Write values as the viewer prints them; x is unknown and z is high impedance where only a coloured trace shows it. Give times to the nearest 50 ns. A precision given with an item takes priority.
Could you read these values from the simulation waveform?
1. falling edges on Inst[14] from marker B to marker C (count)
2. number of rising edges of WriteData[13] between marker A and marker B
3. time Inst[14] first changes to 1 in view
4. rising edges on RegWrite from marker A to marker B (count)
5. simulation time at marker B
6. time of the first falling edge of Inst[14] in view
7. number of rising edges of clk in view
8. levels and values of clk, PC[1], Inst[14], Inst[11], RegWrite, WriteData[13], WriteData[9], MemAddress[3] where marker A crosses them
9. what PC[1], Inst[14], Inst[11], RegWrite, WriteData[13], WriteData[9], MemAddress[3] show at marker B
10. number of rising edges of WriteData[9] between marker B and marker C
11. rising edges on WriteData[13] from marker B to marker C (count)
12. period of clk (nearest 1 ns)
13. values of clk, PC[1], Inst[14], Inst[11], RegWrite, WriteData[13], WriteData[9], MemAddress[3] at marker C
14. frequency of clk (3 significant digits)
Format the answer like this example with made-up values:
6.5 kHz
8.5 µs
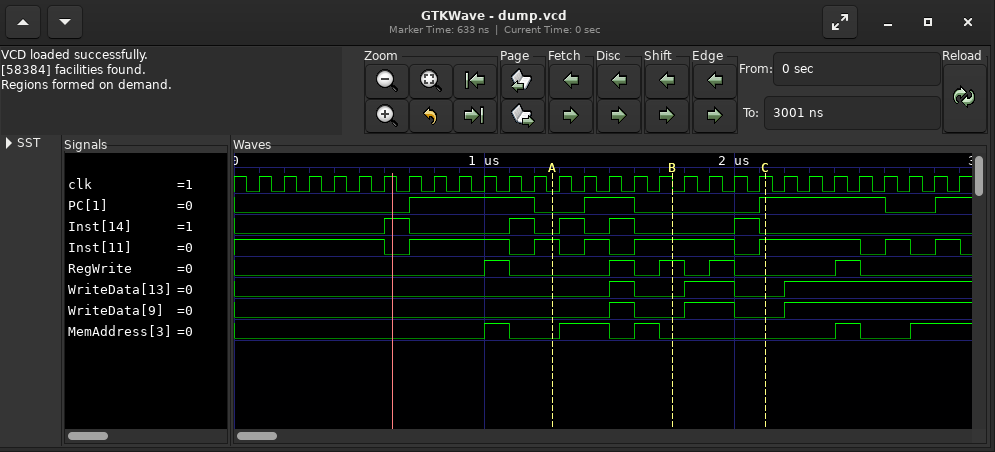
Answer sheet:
1
1
600 ns
2
1750 ns
700 ns
29
clk=0, PC[1]=0, Inst[14]=0, Inst[11]=1, RegWrite=0, WriteData[13]=0, WriteData[9]=0, MemAddress[3]=0
PC[1]=0, Inst[14]=0, Inst[11]=1, RegWrite=1, WriteData[13]=0, WriteData[9]=0, MemAddress[3]=0
1
1
100 ns
clk=1, PC[1]=1, Inst[14]=0, Inst[11]=1, RegWrite=0, WriteData[13]=0, WriteData[9]=0, MemAddress[3]=0
10.0 MHz
